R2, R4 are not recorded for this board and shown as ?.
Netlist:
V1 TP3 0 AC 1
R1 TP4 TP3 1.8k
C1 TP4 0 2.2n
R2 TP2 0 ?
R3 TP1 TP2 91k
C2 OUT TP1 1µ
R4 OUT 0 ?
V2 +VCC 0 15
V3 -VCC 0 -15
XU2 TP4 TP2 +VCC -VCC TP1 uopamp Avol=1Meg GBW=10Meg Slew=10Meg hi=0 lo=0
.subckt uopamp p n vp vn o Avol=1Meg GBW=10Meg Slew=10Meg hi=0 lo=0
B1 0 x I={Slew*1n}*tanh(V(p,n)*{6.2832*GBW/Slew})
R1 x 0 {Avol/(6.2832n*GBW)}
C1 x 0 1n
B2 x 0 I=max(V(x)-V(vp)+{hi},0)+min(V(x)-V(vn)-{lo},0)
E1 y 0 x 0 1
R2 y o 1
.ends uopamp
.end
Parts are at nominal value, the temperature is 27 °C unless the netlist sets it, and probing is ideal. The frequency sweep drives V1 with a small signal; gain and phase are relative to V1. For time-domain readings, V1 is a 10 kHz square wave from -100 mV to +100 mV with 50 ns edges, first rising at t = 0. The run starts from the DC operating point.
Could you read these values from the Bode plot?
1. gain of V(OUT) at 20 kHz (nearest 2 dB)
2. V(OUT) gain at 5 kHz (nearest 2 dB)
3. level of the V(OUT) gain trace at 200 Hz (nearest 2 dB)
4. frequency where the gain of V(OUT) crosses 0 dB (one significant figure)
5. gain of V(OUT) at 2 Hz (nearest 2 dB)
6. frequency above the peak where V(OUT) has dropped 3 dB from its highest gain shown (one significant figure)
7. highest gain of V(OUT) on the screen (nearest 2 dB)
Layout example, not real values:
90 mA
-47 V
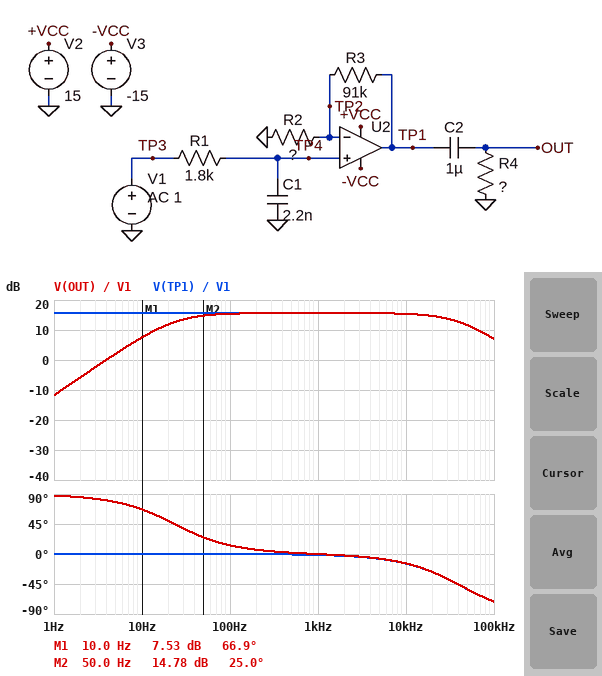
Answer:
14 dB
16 dB
16 dB
4 Hz
-6 dB
40 kHz
16 dB
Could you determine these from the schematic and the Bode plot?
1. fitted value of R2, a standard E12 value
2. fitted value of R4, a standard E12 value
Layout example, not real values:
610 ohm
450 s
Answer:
18 kΩ
6.8 kΩ
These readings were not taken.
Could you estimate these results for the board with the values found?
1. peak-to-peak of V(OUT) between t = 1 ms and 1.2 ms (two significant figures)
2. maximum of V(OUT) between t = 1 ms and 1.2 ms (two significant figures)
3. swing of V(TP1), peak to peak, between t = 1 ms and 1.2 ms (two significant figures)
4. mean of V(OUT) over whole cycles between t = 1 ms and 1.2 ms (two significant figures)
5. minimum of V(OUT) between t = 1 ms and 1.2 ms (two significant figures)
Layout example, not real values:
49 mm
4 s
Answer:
1.2 V
1.1 V
1.2 V
520 mV
-98 mV
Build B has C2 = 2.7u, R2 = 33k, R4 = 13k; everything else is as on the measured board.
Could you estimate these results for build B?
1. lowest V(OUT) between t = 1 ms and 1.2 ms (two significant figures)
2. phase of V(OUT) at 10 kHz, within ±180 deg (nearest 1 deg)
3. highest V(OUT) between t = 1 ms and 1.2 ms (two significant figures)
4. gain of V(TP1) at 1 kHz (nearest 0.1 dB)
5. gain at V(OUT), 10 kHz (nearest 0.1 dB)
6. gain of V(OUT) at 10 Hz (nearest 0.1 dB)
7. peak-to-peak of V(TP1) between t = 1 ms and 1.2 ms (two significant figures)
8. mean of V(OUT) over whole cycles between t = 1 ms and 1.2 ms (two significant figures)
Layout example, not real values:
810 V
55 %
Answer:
-13 mV
-14 deg
740 mV
11.5 dB
11.2 dB
10.7 dB
750 mV
360 mV
